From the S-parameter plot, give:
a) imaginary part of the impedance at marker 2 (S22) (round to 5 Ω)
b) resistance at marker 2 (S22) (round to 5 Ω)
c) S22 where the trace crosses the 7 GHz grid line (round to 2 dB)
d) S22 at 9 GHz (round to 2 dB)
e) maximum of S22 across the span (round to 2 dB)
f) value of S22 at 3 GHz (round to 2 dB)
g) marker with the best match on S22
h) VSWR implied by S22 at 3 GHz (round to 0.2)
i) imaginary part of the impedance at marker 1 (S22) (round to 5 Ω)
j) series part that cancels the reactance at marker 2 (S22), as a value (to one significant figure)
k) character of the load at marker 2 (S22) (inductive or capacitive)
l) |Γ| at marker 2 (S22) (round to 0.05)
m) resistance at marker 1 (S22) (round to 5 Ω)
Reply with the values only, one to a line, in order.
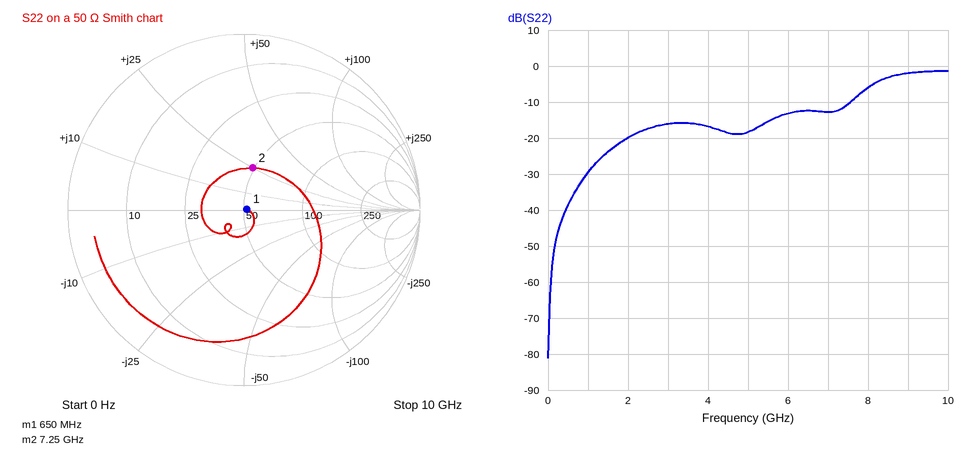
+25 Ω
50 Ω
-12 dB
-2 dB
-2 dB
-16 dB
marker 1
1.4
0 Ω
900 fF
inductive
0.25
50 Ω
